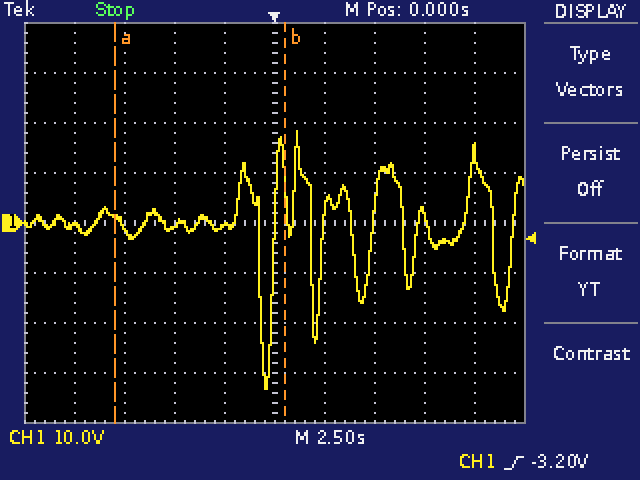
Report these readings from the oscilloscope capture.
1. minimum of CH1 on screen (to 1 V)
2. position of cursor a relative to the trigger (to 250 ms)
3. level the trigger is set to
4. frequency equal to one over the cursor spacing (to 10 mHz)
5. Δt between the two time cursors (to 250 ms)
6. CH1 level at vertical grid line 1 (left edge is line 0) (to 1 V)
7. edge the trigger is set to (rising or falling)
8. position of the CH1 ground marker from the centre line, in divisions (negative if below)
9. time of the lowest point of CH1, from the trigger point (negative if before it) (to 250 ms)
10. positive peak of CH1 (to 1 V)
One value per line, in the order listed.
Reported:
-33 V
-8.00 s
-3.20 V
120 mHz
8.50 s
-1 V
rising
0.0 div
-500 ms
18 V
